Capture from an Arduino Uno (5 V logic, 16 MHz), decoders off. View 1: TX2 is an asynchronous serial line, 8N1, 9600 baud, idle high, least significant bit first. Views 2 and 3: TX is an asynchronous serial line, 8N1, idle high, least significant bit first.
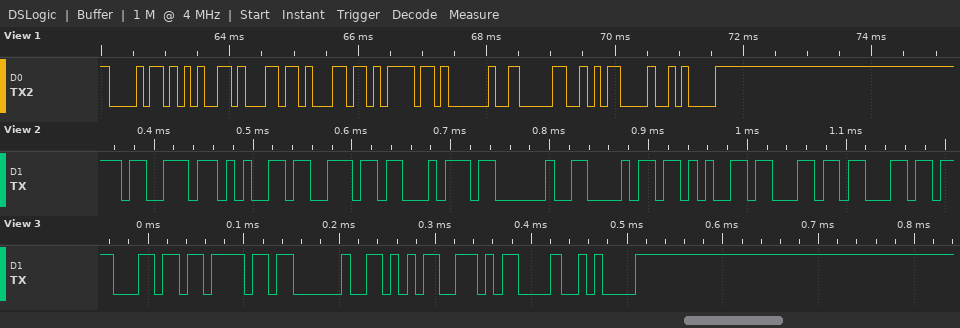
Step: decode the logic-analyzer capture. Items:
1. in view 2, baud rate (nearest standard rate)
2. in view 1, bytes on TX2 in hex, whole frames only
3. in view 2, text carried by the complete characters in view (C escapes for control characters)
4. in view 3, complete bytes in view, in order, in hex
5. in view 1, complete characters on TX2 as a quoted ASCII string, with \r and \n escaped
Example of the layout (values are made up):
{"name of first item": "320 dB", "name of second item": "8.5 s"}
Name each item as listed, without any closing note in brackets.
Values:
{"in view 2, baud rate": "115200 baud", "in view 1, bytes on TX2 in hex, whole frames only": "0x68 0x65 0x6C 0x6C 0x6F 0x20 0x30 0x0D 0x0A", "in view 2, text carried by the complete characters in view": "\"sent hell\"", "in view 3, complete bytes in view, in order, in hex": "6C 6F 20 35 0D 0A", "in view 1, complete characters on TX2 as a quoted ASCII string, with \\r and \\n escaped": "\"hello 0\\r\\n\""}
